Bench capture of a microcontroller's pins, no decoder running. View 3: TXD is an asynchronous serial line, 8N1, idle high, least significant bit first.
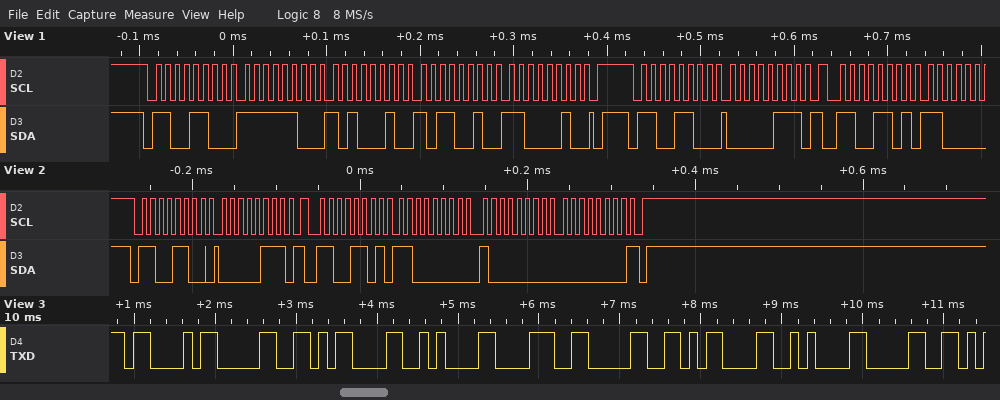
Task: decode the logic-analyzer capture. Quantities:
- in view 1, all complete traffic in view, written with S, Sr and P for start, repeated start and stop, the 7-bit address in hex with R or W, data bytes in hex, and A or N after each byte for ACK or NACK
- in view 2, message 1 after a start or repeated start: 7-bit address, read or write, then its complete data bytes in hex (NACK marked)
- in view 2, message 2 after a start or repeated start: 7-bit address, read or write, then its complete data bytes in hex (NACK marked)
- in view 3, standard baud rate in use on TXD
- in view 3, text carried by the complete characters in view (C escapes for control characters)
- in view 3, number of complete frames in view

S 66W A FC A A2 A B2 A C2 A P S 66W A 07 A Sr 66R A
0x66 write: 07
0x66 read: C0 80 00 NACK
9600 baud
"C0\r\n80\r\n0"
9
